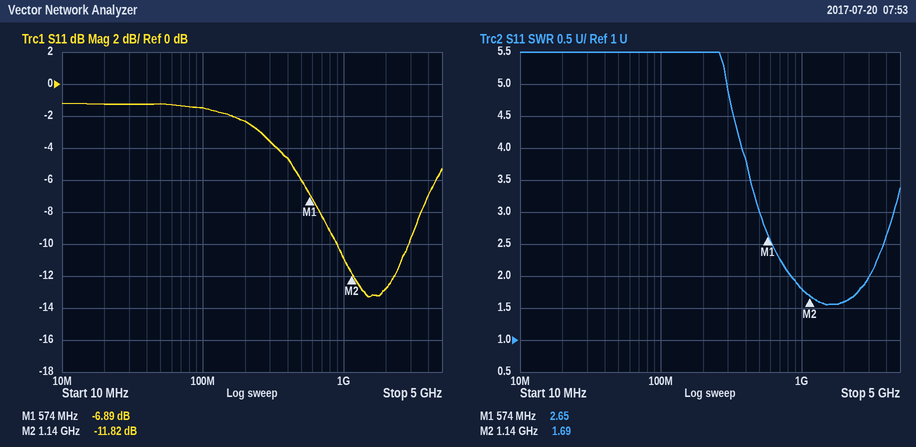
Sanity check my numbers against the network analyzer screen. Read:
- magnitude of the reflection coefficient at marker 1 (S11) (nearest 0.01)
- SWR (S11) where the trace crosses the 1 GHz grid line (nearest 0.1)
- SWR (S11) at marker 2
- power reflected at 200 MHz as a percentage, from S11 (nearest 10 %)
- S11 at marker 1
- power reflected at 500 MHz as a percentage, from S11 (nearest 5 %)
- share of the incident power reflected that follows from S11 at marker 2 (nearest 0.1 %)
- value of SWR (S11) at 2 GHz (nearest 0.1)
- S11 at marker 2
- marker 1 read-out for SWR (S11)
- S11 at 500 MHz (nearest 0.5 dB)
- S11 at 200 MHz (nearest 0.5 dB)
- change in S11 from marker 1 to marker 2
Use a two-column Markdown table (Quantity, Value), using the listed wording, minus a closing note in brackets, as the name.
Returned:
| Quantity | Value |
|---|---|
| magnitude of the reflection coefficient at marker 1 (S11) | 0.45 |
| SWR (S11) where the trace crosses the 1 GHz grid line | 1.8 |
| SWR (S11) at marker 2 | 1.69 |
| power reflected at 200 MHz as a percentage, from S11 | 60 % |
| S11 at marker 1 | -6.89 dB |
| power reflected at 500 MHz as a percentage, from S11 | 25 % |
| share of the incident power reflected that follows from S11 at marker 2 | 6.6 % |
| value of SWR (S11) at 2 GHz | 1.6 |
| S11 at marker 2 | -11.82 dB |
| marker 1 read-out for SWR | 2.65 |
| S11 at 500 MHz | -6.0 dB |
| S11 at 200 MHz | -2.5 dB |
| change in S11 from marker 1 to marker 2 | -4.93 dB |
